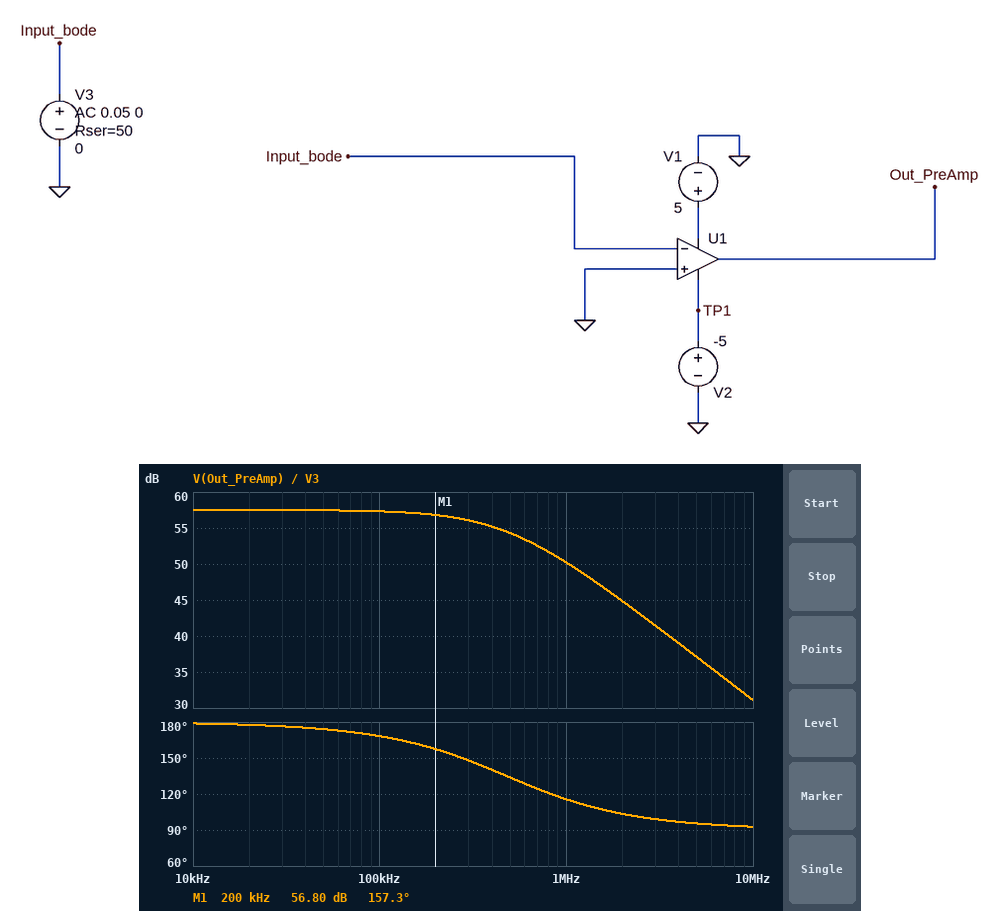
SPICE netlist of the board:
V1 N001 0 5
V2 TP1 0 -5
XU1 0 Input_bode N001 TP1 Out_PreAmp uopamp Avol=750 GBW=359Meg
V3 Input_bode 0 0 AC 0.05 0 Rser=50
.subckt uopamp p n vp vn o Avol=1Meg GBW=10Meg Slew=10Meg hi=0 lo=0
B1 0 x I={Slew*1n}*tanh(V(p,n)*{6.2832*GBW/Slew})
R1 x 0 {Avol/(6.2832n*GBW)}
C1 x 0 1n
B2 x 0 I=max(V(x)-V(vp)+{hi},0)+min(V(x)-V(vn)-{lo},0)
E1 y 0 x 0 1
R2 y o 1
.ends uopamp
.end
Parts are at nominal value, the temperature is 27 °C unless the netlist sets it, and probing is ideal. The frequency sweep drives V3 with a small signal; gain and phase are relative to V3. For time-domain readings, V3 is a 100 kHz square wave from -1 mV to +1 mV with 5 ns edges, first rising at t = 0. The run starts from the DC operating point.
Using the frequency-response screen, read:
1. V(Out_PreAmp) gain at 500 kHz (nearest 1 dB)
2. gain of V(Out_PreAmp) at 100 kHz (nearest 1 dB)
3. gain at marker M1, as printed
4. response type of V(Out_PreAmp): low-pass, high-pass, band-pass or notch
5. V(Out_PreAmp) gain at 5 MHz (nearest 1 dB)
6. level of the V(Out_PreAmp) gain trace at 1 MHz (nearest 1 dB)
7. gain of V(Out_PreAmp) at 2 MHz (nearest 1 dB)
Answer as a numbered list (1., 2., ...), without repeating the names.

1. 54 dB
2. 57 dB
3. 56.80 dB
4. low-pass
5. 37 dB
6. 50 dB
7. 45 dB
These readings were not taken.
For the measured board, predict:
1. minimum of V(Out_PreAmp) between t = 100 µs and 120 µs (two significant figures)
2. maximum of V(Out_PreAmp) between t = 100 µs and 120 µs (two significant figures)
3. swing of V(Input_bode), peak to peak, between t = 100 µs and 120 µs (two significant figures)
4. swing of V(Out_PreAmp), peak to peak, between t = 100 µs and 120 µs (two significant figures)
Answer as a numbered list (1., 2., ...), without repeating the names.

1. -740 mV
2. 740 mV
3. 2.0 mV
4. 1.5 V
